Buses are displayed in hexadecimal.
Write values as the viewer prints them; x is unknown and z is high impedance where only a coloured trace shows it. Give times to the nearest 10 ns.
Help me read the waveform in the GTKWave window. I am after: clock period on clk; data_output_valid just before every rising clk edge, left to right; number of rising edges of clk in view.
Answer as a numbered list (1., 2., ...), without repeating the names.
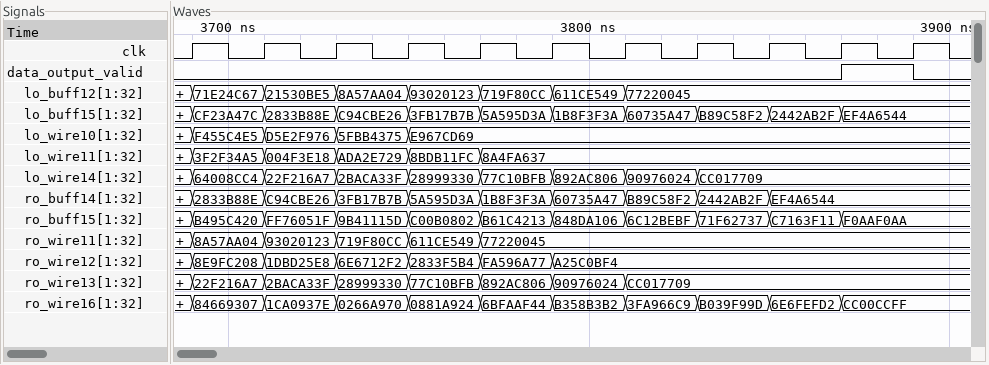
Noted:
1. 20 ns
2. 0 0 0 0 0 0 0 0 0 0 1
3. 11
